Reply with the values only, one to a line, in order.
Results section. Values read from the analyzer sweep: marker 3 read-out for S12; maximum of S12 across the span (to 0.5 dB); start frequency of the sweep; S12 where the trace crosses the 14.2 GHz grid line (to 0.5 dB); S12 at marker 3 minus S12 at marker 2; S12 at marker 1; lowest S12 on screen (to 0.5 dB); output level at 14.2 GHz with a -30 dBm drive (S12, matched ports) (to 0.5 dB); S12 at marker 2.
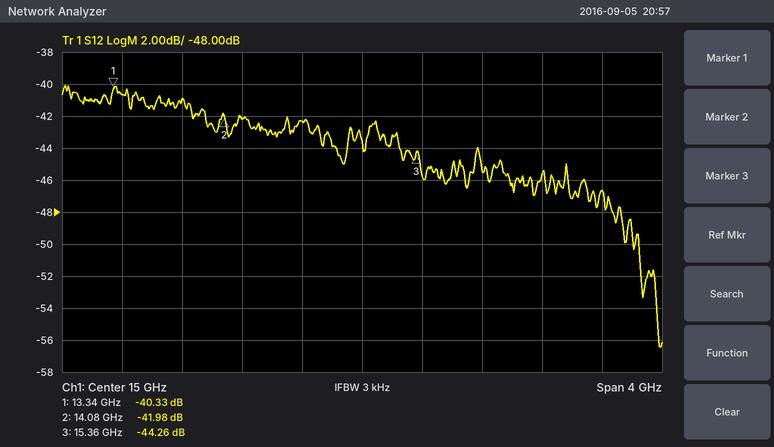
-44.26 dB
-40.0 dB
13 GHz
-42.0 dB
-2.28 dB
-40.33 dB
-56.5 dB
-72.0 dBm
-41.98 dB
